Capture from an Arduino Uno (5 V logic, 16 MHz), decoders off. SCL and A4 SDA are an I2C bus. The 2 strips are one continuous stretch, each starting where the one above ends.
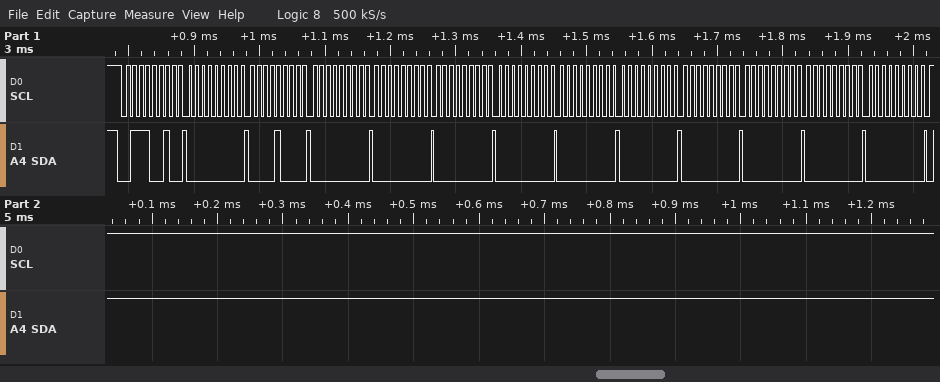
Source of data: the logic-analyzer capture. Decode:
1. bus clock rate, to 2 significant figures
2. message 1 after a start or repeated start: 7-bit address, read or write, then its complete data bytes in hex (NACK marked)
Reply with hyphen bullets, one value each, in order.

- 100 kHz
- 0x39 write: 00 08 00 00 00 00 00 00 00 00 00 00
